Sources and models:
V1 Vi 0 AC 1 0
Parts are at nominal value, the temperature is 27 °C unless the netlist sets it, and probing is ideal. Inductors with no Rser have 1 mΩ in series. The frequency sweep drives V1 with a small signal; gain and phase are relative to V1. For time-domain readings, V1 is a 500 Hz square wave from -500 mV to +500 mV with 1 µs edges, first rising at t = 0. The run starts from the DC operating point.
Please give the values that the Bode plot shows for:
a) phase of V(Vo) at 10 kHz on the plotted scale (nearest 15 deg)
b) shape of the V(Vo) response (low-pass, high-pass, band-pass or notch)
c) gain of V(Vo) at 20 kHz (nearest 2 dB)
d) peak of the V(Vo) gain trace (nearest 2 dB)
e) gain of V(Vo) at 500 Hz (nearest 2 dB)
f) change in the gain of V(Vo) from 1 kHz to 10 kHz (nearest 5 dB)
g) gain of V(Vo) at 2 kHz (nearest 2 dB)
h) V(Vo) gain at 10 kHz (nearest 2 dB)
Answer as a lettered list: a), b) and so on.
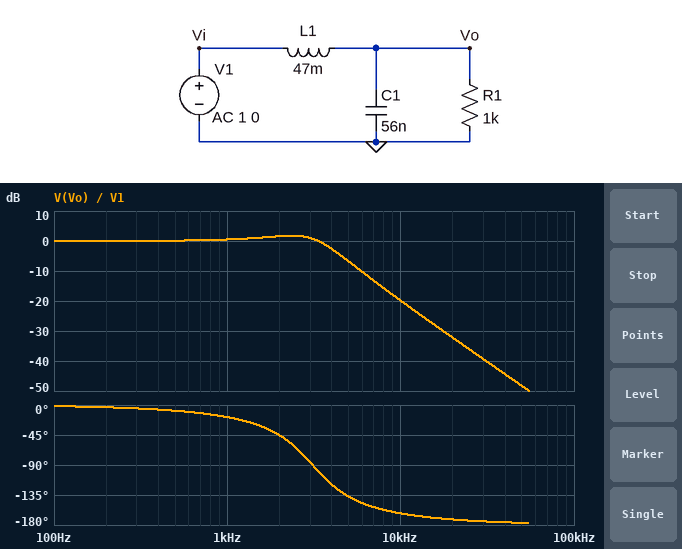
a) -165 deg
b) low-pass
c) -32 dB
d) 2 dB
e) 0 dB
f) -20 dB
g) 2 dB
h) -20 dB
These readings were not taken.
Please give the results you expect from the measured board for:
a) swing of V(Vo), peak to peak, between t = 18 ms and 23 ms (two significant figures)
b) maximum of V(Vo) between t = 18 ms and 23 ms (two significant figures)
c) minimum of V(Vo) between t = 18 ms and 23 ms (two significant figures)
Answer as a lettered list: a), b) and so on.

a) 1.4 V
b) 700 mV
c) -700 mV
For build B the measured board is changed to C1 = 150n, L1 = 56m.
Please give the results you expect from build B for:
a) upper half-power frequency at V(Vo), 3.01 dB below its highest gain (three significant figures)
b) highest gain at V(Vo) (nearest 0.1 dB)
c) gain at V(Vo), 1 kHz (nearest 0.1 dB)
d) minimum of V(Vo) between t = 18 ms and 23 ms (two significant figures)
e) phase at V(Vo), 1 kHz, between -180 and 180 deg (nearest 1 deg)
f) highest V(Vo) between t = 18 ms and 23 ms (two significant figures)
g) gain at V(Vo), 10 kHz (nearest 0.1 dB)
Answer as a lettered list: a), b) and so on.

a) 2.05 kHz
b) 4.7 dB
c) 2.4 dB
d) -880 mV
e) -28 deg
f) 880 mV
g) -30.2 dB
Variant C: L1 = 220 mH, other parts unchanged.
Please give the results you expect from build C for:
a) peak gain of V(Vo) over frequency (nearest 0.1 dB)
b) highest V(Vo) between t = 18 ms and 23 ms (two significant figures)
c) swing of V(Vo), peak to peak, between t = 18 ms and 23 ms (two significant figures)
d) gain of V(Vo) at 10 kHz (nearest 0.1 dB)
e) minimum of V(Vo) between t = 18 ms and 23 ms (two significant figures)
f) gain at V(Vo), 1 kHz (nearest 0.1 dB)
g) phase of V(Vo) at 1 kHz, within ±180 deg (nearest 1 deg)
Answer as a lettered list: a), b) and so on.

a) 0 dB
b) 500 mV
c) 1.0 V
d) -33.9 dB
e) -500 mV
f) -3.4 dB
g) -70 deg
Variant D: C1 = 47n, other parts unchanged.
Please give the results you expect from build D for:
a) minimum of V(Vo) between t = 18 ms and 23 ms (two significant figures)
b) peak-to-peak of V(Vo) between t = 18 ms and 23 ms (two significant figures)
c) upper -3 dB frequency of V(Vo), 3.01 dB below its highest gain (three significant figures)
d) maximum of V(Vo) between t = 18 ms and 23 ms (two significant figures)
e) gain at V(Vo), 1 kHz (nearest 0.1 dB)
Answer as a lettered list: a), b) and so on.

a) -660 mV
b) 1.3 V
c) 3.96 kHz
d) 660 mV
e) 0.4 dB
